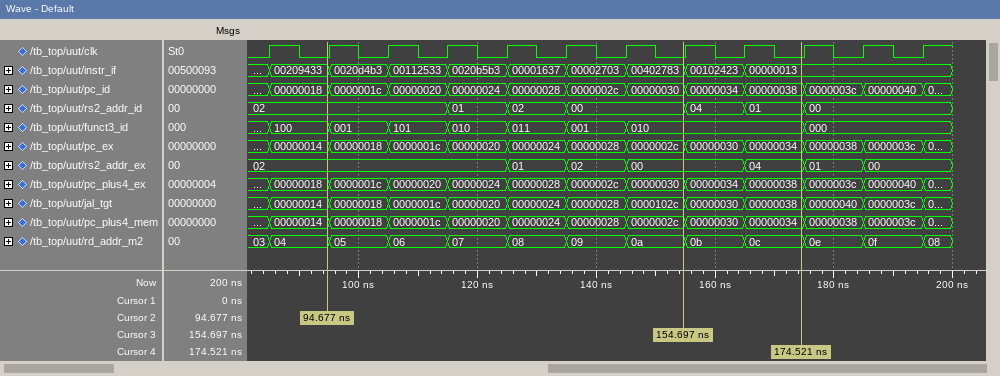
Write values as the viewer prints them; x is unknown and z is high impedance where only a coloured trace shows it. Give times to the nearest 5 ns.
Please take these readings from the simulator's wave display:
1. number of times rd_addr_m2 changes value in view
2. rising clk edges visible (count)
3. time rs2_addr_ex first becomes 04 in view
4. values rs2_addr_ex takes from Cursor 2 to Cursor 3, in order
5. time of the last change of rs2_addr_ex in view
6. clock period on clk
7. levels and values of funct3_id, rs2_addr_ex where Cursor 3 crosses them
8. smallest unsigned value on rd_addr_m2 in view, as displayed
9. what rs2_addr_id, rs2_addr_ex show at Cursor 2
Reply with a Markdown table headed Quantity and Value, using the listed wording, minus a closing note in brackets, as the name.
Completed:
| Quantity | Value |
|---|---|
| number of times rd_addr_m2 changes value in view | 12 |
| rising clk edges visible | 12 |
| time rs2_addr_ex first becomes 04 in view | 165 ns |
| values rs2_addr_ex takes from Cursor 2 to Cursor 3, in order | 02, 01, 02, 00 |
| time of the last change of rs2_addr_ex in view | 185 ns |
| clock period on clk | 10 ns |
| levels and values of funct3_id, rs2_addr_ex where Cursor 3 crosses them | funct3_id=010, rs2_addr_ex=00 |
| smallest unsigned value on rd_addr_m2 in view, as displayed | 03 |
| what rs2_addr_id, rs2_addr_ex show at Cursor 2 | rs2_addr_id=02, rs2_addr_ex=02 |
